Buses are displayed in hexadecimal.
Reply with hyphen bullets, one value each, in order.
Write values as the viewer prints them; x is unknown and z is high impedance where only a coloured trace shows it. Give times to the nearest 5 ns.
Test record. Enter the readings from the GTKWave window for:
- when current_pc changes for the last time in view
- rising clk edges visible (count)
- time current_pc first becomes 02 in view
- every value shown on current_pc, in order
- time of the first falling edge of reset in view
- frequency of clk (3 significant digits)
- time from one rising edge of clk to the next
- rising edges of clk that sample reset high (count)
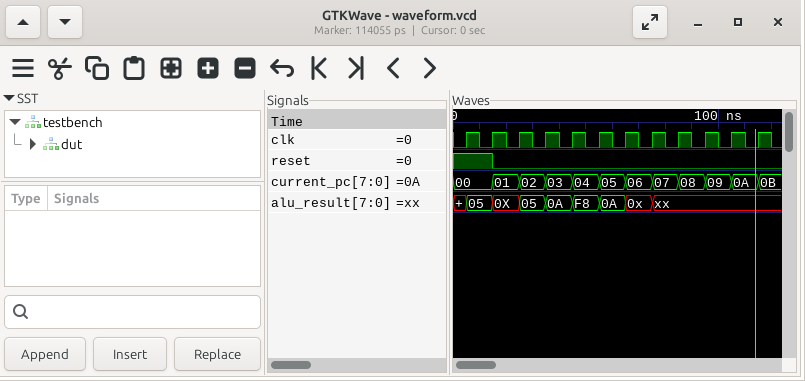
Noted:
- 115 ns
- 12
- 25 ns
- 00, 01, 02, 03, 04, 05, 06, 07, 08, 09, 0A, 0B
- 15 ns
- 100 MHz
- 10 ns
- 2
